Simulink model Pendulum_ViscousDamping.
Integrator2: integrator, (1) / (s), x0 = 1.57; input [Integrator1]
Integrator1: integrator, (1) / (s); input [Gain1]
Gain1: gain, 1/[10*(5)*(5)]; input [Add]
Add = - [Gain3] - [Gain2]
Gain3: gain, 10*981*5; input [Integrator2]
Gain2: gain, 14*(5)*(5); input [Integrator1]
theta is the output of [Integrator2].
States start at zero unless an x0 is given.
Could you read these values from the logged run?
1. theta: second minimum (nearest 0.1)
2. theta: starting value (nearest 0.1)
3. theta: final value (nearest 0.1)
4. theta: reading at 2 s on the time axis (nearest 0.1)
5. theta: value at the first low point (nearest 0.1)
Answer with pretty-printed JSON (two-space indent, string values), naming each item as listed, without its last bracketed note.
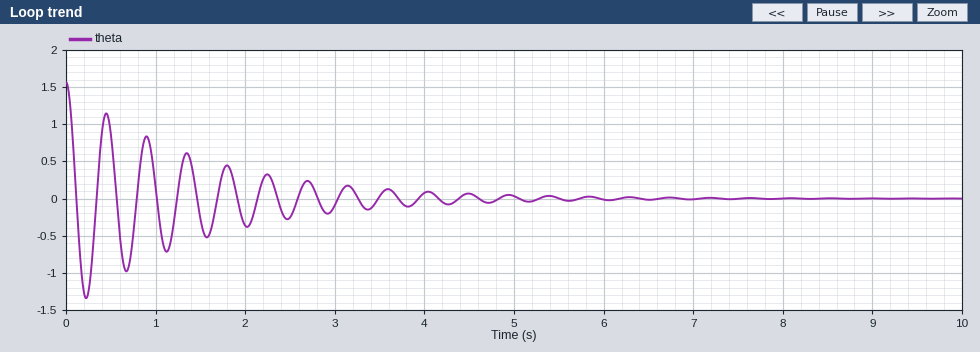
{
  "theta: second minimum": "-1.0",
  "theta: starting value": "1.6",
  "theta: final value": "0.0",
  "theta: reading at 2 s on the time axis": "-0.4",
  "theta: value at the first low point": "-1.3"
}
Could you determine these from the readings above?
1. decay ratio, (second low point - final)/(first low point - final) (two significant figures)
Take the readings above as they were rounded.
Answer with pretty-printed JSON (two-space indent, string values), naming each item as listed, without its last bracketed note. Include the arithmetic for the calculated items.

{
  "decay ratio, (second low point - final)/(first low point - final)": "(-1 - 0) / (-1.3 - 0) = 0.77"
}
